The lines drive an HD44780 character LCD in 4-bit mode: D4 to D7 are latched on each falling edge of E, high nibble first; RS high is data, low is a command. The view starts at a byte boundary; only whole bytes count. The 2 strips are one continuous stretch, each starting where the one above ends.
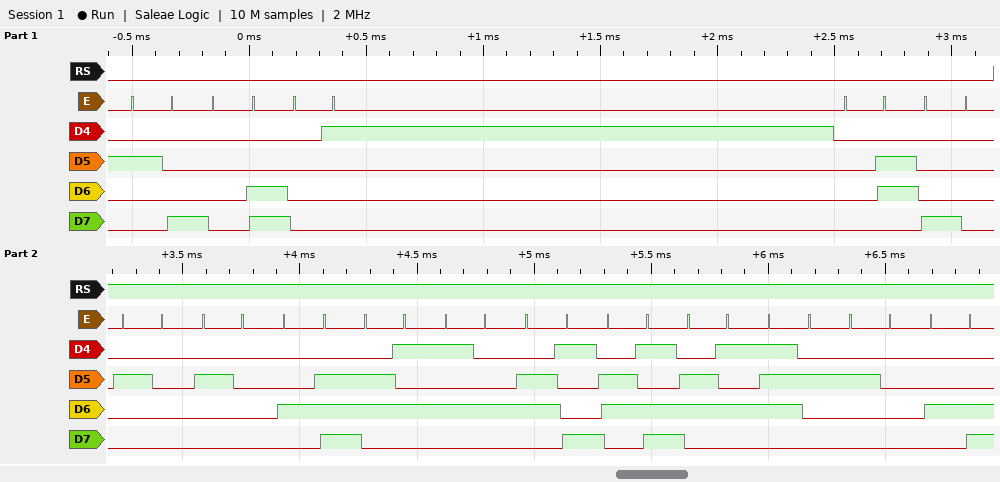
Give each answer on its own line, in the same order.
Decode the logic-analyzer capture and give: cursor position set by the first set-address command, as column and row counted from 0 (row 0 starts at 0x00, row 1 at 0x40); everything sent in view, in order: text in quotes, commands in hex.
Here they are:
column 0, row 0
0x28 0x0C 0x01 0x06 0x80 "  NeTimer L"
